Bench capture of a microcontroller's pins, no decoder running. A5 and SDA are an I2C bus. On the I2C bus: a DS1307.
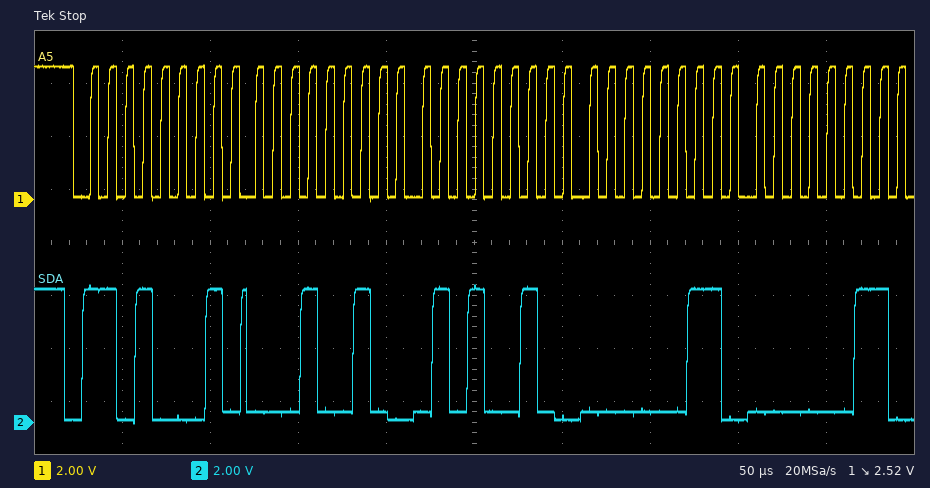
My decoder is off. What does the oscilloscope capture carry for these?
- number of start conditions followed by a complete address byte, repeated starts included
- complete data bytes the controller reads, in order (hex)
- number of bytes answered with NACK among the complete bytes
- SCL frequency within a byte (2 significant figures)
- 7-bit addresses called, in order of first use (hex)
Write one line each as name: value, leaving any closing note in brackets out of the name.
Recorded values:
number of start conditions followed by a complete address byte, repeated starts included: 1
complete data bytes the controller reads, in order: 12 52 03 03
number of bytes answered with NACK among the complete bytes: 0
SCL frequency within a byte: 100 kHz
7-bit addresses called, in order of first use: 0x68
